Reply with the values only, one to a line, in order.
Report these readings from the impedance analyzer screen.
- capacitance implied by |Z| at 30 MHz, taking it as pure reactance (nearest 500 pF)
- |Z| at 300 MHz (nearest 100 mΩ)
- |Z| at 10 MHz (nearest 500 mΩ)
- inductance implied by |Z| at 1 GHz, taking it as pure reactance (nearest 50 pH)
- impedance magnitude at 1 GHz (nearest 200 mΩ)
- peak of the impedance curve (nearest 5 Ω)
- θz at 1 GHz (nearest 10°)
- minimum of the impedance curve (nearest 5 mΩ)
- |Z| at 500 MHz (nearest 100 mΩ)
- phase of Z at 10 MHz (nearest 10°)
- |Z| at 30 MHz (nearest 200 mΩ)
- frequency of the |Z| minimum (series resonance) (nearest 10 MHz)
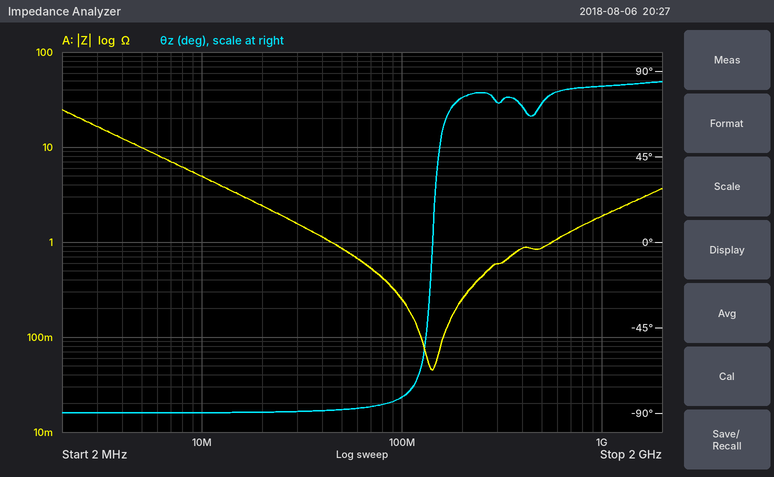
3.5 nF
600 mΩ
5.0 Ω
300 pH
1.8 Ω
25 Ω
80°
45 mΩ
900 mΩ
-90°
1.6 Ω
140 MHz
